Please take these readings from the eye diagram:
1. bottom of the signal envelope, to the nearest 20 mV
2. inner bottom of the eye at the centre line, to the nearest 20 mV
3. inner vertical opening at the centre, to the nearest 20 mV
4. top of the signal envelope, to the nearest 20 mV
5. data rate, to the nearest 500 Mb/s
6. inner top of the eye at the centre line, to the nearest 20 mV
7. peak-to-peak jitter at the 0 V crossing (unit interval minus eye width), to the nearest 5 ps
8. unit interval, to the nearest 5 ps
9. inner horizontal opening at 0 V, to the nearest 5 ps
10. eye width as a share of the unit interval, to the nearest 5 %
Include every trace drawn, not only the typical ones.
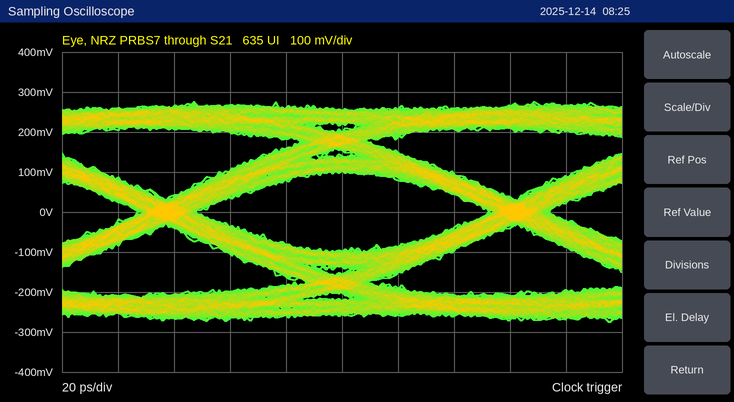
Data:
-280 mV
-100 mV
200 mV
280 mV
8.0 Gb/s
100 mV
20 ps
125 ps
105 ps
85 %
